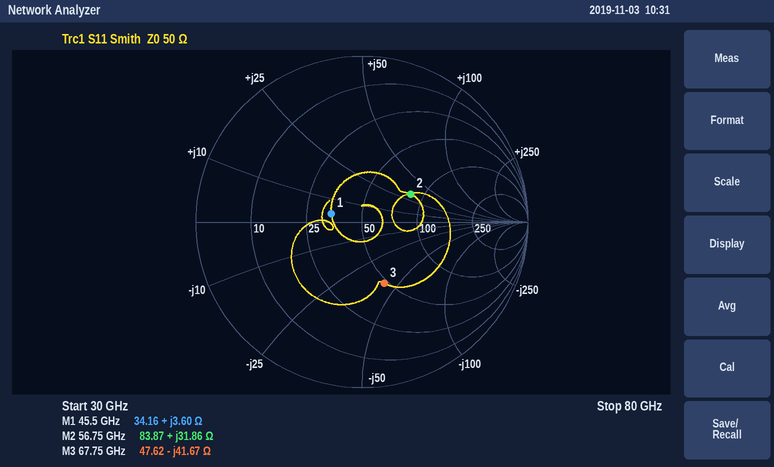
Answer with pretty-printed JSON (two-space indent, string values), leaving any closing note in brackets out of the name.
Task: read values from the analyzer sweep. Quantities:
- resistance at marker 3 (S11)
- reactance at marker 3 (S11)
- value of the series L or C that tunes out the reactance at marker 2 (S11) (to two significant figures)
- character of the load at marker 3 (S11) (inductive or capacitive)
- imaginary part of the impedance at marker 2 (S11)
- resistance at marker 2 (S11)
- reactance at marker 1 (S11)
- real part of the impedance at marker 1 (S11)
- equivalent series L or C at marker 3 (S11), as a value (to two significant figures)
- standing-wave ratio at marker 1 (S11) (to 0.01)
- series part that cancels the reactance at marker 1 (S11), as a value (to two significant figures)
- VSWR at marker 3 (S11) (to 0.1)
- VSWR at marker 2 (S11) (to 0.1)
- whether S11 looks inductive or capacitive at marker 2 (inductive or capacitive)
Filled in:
{
  "resistance at marker 3": "47.62 Ω",
  "reactance at marker 3": "-41.67 Ω",
  "value of the series L or C that tunes out the reactance at marker 2 (S11)": "88 fF",
  "character of the load at marker 3 (S11)": "capacitive",
  "imaginary part of the impedance at marker 2": "+31.86 Ω",
  "resistance at marker 2": "83.87 Ω",
  "reactance at marker 1": "+3.60 Ω",
  "real part of the impedance at marker 1": "34.16 Ω",
  "equivalent series L or C at marker 3 (S11), as a value": "56 fF",
  "standing-wave ratio at marker 1 (S11)": "1.48",
  "series part that cancels the reactance at marker 1 (S11), as a value": "970 fF",
  "VSWR at marker 3 (S11)": "2.3",
  "VSWR at marker 2 (S11)": "2.0",
  "whether S11 looks inductive or capacitive at marker 2": "inductive"
}
